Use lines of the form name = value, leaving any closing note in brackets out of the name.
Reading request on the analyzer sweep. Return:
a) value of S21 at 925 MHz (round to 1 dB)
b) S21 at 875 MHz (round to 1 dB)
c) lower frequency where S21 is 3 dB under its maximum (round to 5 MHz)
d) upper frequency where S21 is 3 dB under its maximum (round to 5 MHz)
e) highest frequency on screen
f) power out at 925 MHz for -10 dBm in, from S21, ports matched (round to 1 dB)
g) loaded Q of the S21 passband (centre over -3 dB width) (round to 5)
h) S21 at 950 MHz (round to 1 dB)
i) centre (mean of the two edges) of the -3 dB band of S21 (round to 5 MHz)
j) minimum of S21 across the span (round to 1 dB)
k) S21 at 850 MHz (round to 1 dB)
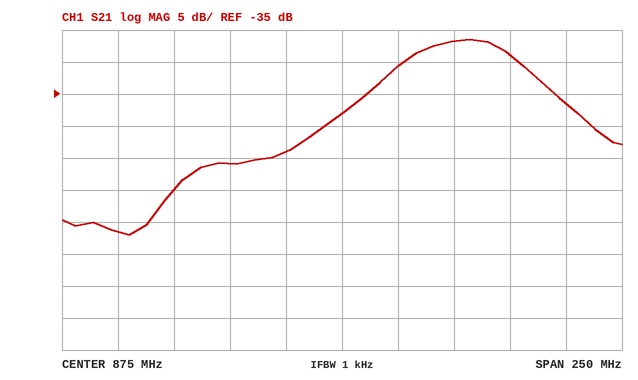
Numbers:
value of S21 at 925 MHz = -27 dB
S21 at 875 MHz = -38 dB
lower frequency where S21 is 3 dB under its maximum = 905 MHz
upper frequency where S21 is 3 dB under its maximum = 950 MHz
highest frequency on screen = 1 GHz
power out at 925 MHz for -10 dBm in, from S21, ports matched = -37 dBm
loaded Q of the S21 passband (centre over -3 dB width) = 20
S21 at 950 MHz = -29 dB
centre (mean of the two edges) of the -3 dB band of S21 = 930 MHz
minimum of S21 across the span = -57 dB
S21 at 850 MHz = -44 dB
